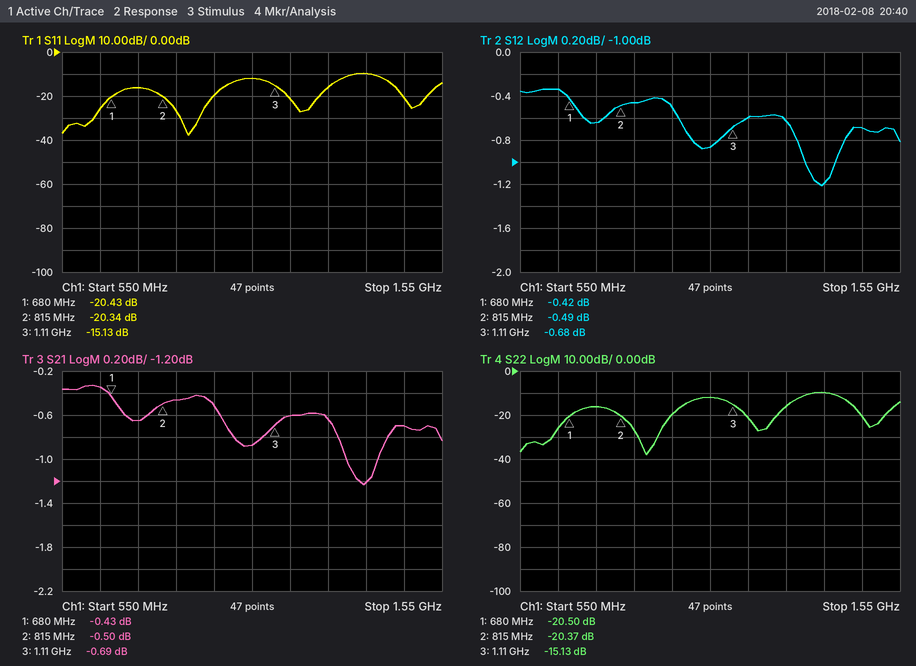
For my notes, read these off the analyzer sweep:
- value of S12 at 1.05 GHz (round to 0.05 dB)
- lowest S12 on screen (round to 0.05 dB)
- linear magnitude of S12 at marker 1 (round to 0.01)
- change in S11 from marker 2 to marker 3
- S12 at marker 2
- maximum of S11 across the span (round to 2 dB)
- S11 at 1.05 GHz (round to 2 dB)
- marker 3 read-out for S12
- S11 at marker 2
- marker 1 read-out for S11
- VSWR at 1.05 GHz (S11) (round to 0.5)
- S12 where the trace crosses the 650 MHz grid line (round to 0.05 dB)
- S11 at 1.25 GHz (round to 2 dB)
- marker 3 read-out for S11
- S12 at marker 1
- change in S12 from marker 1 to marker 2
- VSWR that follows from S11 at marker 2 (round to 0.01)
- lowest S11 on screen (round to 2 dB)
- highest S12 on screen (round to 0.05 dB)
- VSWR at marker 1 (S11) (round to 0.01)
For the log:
-0.85 dB
-1.20 dB
0.95
5.21 dB
-0.49 dB
-10 dB
-12 dB
-0.68 dB
-20.34 dB
-20.43 dB
1.5
-0.35 dB
-16 dB
-15.13 dB
-0.42 dB
-0.07 dB
1.21
-38 dB
-0.35 dB
1.21
